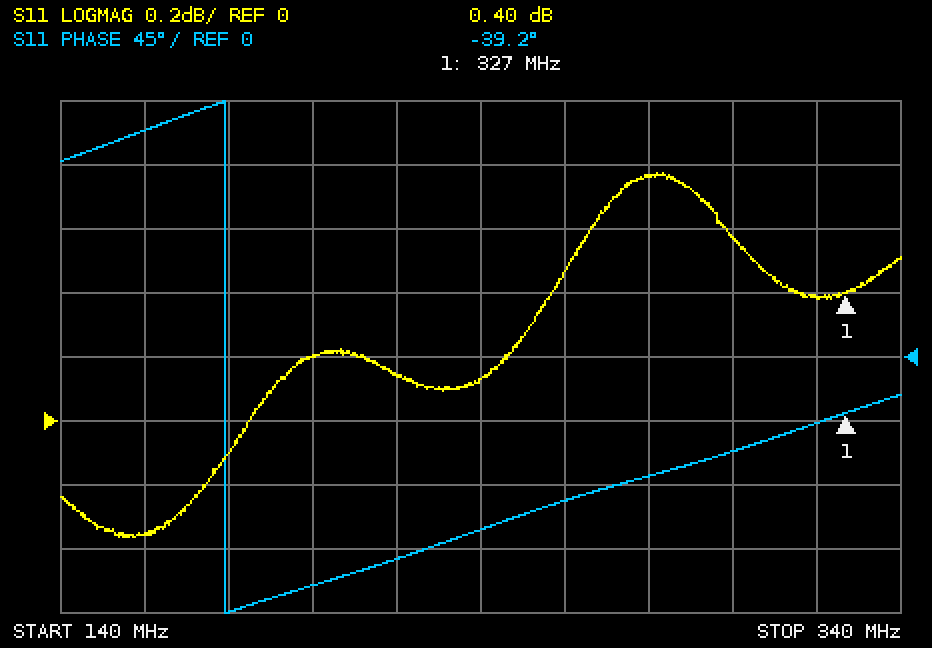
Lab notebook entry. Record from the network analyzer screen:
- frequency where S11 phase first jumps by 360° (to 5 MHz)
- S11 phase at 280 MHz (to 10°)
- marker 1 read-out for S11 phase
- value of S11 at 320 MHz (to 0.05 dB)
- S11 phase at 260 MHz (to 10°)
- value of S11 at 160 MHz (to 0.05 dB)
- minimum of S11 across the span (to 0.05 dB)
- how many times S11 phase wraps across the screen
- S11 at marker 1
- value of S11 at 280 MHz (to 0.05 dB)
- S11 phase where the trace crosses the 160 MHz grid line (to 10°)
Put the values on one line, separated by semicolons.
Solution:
180 MHz; -80°; -39.2°; 0.40 dB; -100°; -0.35 dB; -0.35 dB; 1; 0.40 dB; 0.75 dB; 160°
